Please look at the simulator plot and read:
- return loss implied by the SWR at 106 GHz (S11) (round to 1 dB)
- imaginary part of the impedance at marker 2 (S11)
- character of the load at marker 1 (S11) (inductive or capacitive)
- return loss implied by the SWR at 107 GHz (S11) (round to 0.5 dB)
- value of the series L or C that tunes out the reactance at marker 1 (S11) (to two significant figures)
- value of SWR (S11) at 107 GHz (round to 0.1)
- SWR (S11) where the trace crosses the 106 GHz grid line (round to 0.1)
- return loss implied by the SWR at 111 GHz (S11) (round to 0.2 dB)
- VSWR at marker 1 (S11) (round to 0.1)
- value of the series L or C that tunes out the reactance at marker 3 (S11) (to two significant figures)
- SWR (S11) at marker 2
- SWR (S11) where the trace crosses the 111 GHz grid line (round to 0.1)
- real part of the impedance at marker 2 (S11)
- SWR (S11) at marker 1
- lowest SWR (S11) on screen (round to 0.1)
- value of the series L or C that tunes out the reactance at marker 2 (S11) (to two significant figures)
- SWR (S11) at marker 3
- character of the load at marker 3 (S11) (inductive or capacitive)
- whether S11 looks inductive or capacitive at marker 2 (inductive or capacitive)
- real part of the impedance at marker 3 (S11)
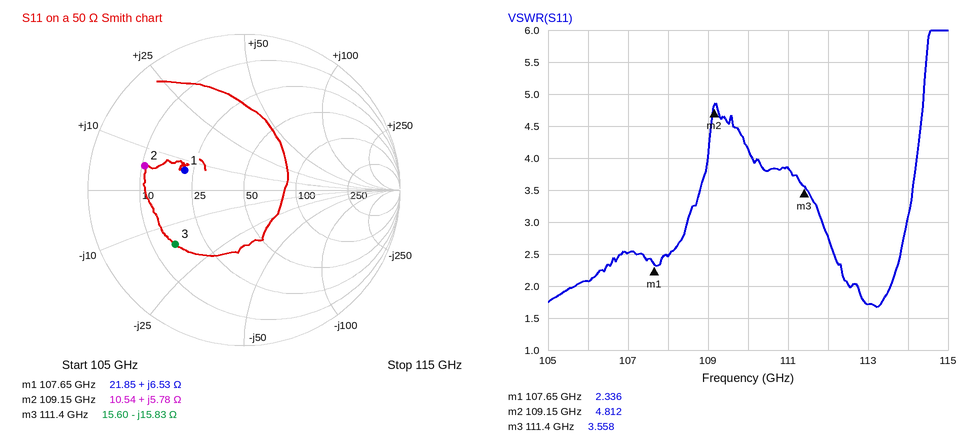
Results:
9 dB
+5.78 Ω
inductive
7.5 dB
230 fF
2.5
2.1
4.6 dB
2.3
23 pH
4.812
3.8
10.54 Ω
2.336
1.7
250 fF
3.558
capacitive
inductive
15.60 Ω
